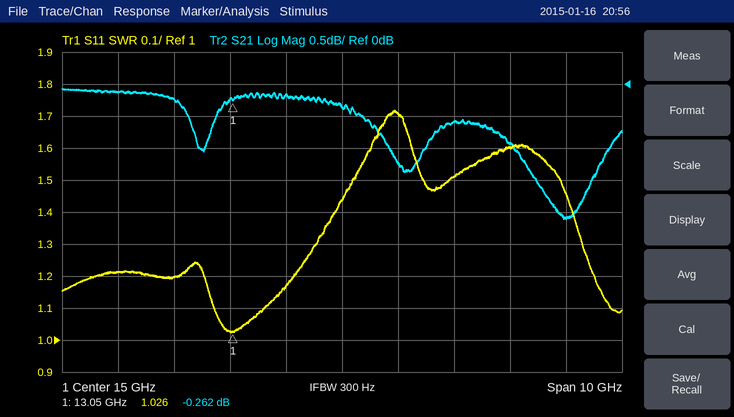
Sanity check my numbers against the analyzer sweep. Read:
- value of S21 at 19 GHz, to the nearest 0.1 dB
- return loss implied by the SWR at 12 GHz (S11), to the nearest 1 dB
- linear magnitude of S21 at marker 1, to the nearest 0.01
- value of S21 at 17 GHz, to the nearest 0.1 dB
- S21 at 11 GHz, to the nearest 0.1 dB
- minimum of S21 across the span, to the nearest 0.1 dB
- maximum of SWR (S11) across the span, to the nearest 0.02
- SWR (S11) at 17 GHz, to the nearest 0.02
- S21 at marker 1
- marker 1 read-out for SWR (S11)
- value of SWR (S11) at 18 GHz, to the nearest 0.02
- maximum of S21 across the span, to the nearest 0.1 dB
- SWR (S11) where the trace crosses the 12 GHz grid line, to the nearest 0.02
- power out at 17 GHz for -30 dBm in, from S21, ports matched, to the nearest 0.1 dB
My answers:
-2.1 dB
21 dB
0.97
-0.6 dB
-0.1 dB
-2.1 dB
1.72
1.52
-0.262 dB
1.026
1.60
-0.1 dB
1.20
-30.6 dBm
